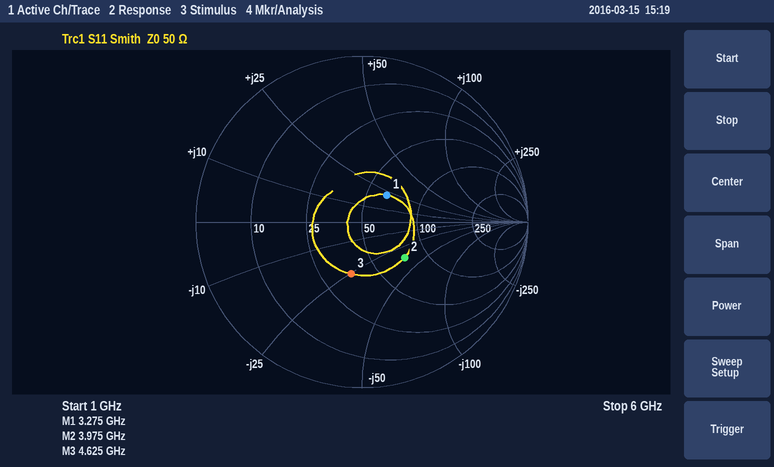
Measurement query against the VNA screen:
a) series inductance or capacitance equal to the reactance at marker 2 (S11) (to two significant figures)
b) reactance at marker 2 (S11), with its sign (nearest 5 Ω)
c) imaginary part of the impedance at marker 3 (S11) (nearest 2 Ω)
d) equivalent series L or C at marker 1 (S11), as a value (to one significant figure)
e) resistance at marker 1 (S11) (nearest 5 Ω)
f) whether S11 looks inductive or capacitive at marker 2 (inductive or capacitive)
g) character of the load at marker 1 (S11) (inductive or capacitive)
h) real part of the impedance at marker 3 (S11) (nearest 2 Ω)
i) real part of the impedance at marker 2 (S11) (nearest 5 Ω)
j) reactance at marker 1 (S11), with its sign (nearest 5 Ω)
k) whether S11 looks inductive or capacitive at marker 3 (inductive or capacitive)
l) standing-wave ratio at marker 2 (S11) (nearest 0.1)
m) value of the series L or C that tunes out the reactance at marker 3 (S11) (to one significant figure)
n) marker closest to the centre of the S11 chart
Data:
1.1 pF
-35 Ω
-26 Ω
1 nH
65 Ω
capacitive
inductive
36 Ω
75 Ω
+20 Ω
capacitive
2.0
900 pH
marker 1
